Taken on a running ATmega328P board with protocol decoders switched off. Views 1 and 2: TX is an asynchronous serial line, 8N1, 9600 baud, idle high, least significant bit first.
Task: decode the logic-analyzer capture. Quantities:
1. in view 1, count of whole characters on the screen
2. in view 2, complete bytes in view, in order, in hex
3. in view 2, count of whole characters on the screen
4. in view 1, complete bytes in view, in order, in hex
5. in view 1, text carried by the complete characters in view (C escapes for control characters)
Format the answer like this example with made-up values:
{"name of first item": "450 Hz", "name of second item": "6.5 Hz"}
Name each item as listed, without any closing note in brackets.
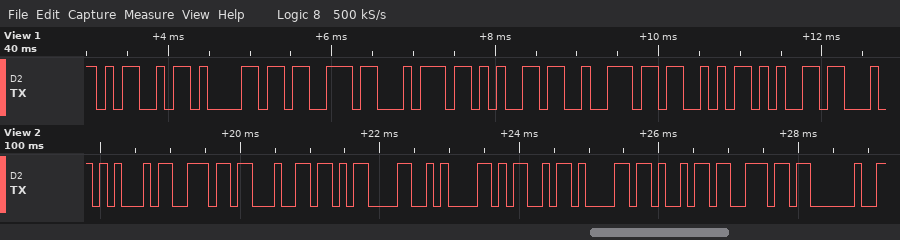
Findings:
{"in view 1, count of whole characters on the screen": "8", "in view 2, complete bytes in view, in order, in hex": "45 6E 64 0D 0A 4D 61 69 6E 20", "in view 2, count of whole characters on the screen": "10", "in view 1, complete bytes in view, in order, in hex": "4D 61 73 74 65 72 53 65", "in view 1, text carried by the complete characters in view": "\"MasterSe\""}
